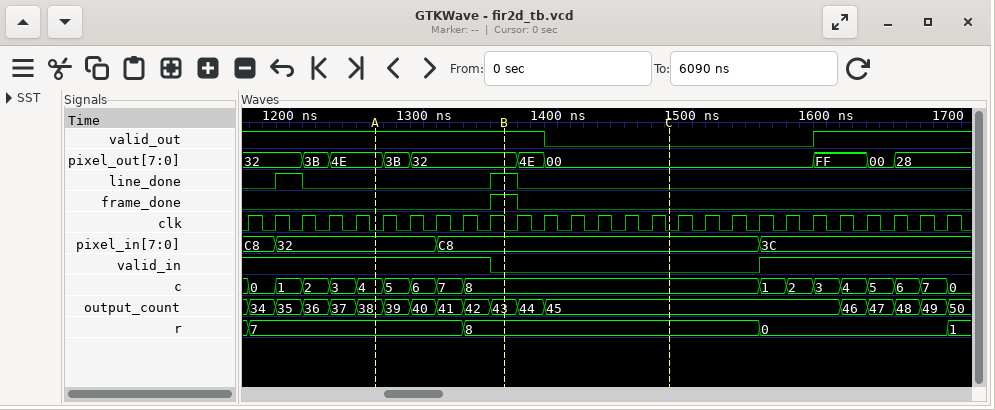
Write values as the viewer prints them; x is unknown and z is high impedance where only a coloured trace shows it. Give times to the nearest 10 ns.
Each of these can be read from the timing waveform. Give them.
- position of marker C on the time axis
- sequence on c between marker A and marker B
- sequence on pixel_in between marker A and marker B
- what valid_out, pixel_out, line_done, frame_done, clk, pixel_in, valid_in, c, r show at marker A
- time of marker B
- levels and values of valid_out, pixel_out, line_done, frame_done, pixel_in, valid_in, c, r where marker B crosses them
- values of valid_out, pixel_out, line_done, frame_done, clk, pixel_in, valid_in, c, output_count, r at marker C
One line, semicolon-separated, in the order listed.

1480 ns; 4, 5, 6, 7, 8; 32, C8; valid_out=1, pixel_out=4E, line_done=0, frame_done=0, clk=0, pixel_in=32, valid_in=1, c=4, r=7; 1360 ns; valid_out=1, pixel_out=32, line_done=1, frame_done=1, pixel_in=C8, valid_in=0, c=8, r=8; valid_out=0, pixel_out=00, line_done=0, frame_done=0, clk=0, pixel_in=C8, valid_in=0, c=8, output_count=45, r=8
